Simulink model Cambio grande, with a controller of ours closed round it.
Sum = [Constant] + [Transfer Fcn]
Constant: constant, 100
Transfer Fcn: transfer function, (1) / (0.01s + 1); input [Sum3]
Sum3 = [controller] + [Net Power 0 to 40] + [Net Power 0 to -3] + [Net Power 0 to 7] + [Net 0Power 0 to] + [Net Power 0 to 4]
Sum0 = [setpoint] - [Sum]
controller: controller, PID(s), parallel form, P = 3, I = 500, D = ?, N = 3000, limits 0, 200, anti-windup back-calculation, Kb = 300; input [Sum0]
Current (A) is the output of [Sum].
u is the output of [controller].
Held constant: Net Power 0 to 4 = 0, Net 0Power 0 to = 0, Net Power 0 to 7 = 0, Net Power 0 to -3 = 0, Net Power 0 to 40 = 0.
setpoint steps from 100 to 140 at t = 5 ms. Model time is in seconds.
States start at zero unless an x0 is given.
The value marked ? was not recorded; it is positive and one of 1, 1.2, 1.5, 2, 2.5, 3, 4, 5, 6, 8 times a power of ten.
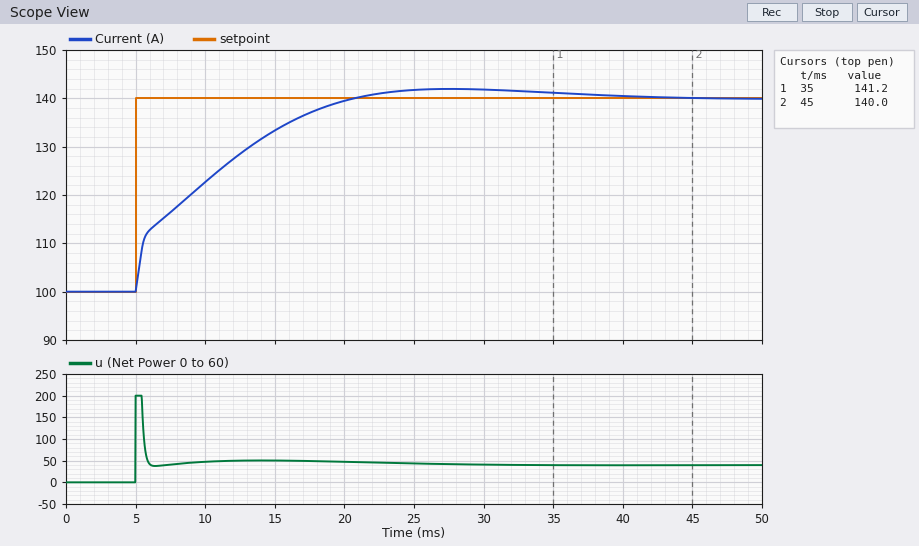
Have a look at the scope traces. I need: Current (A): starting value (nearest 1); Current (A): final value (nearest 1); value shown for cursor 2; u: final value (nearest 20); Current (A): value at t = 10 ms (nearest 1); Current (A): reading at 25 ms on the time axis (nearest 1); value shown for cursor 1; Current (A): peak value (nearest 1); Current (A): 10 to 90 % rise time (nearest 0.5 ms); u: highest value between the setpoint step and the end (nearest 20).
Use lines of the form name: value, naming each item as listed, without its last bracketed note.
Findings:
Current (A): starting value: 100
Current (A): final value: 140
value shown for cursor 2: 140.0
u: final value: 40
Current (A): value at t = 10 ms: 123
Current (A): reading at 25 ms on the time axis: 142
value shown for cursor 1: 141.2
Current (A): peak value: 142
Current (A): 10 to 90 % rise time: 11.5 ms
u: highest value between the setpoint step and the end: 200
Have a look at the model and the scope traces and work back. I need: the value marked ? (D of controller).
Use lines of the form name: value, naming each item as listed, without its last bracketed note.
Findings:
the value marked ?: 0.008
